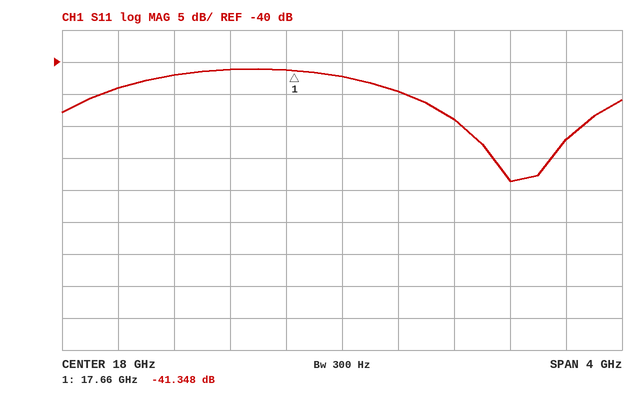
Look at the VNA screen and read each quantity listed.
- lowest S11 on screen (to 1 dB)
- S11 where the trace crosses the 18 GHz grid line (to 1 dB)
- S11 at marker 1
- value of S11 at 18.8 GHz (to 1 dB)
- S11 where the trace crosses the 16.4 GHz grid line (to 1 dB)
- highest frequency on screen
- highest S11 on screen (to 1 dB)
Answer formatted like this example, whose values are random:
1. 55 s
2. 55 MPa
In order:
1. -59 dB
2. -42 dB
3. -41.348 dB
4. -49 dB
5. -44 dB
6. 20 GHz
7. -41 dB
